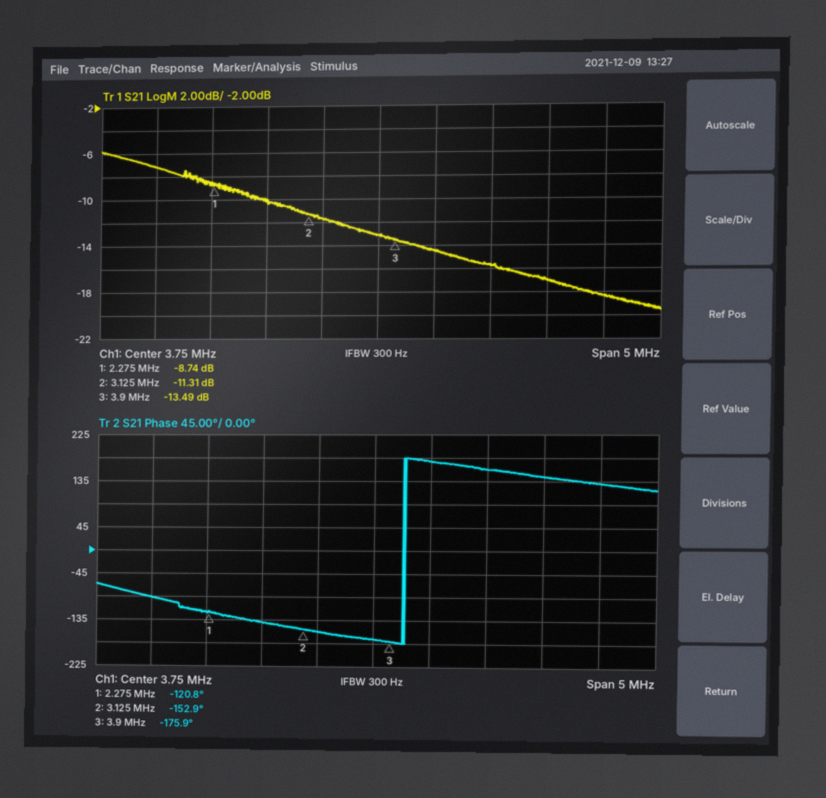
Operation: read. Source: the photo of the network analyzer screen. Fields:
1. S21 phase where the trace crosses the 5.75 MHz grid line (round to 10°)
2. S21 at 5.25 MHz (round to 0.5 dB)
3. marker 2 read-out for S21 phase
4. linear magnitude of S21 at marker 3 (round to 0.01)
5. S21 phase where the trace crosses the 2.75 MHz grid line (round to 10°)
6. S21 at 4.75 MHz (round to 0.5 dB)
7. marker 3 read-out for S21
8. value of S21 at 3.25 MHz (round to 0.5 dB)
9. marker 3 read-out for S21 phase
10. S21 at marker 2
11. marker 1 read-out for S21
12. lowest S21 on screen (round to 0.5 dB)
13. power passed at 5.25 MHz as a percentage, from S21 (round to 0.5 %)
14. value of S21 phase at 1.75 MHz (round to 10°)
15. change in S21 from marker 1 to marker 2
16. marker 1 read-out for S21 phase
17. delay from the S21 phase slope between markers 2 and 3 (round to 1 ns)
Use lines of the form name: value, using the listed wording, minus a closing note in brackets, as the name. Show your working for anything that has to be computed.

S21 phase where the trace crosses the 5.75 MHz grid line: 130°
S21 at 5.25 MHz: -17.0 dB
marker 2 read-out for S21 phase: -152.9°
linear magnitude of S21 at marker 3: 10^(-13.49/20) ≈ 0.21
S21 phase where the trace crosses the 2.75 MHz grid line: -140°
S21 at 4.75 MHz: -15.5 dB
marker 3 read-out for S21: -13.49 dB
value of S21 at 3.25 MHz: -11.5 dB
marker 3 read-out for S21 phase: -175.9°
S21 at marker 2: -11.31 dB
marker 1 read-out for S21: -8.74 dB
lowest S21 on screen: -19.5 dB
power passed at 5.25 MHz as a percentage, from S21: 10^(-17/10) ≈ 2.0 %
value of S21 phase at 1.75 MHz: -90°
change in S21 from marker 1 to marker 2: -11.31 − (-8.74) = -2.57 dB
marker 1 read-out for S21 phase: -120.8°
delay from the S21 phase slope between markers 2 and 3: −(-175.9° − (-152.9°))/(360° × 775 kHz) ≈ 82 ns
